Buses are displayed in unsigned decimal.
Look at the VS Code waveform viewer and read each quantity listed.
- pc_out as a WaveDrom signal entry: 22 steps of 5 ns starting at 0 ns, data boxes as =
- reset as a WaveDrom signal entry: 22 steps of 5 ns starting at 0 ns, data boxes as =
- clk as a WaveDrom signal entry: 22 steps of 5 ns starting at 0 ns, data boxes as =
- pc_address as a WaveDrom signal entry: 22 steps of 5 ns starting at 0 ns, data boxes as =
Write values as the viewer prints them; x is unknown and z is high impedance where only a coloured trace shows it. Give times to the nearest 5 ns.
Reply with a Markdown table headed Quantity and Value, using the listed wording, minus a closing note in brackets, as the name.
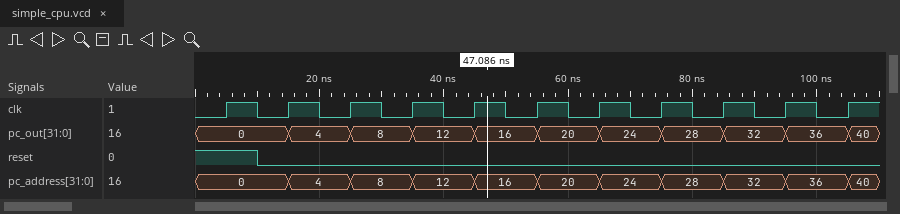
| Quantity | Value |
|---|---|
| pc_out as a WaveDrom signal entry: 22 steps of 5 ns starting at 0 ns, data boxes as = | {name: 'pc_out', wave: '=..=.=.=.=.=.=.=.=.=.=', data: '0 4 8 12 16 20 24 28 32 36 40'} |
| reset as a WaveDrom signal entry: 22 steps of 5 ns starting at 0 ns, data boxes as = | {name: 'reset', wave: '1.0...................'} |
| clk as a WaveDrom signal entry: 22 steps of 5 ns starting at 0 ns, data boxes as = | {name: 'clk', wave: '0101010101010101010101'} |
| pc_address as a WaveDrom signal entry: 22 steps of 5 ns starting at 0 ns, data boxes as = | {name: 'pc_address', wave: '=..=.=.=.=.=.=.=.=.=.=', data: '0 4 8 12 16 20 24 28 32 36 40'} |
